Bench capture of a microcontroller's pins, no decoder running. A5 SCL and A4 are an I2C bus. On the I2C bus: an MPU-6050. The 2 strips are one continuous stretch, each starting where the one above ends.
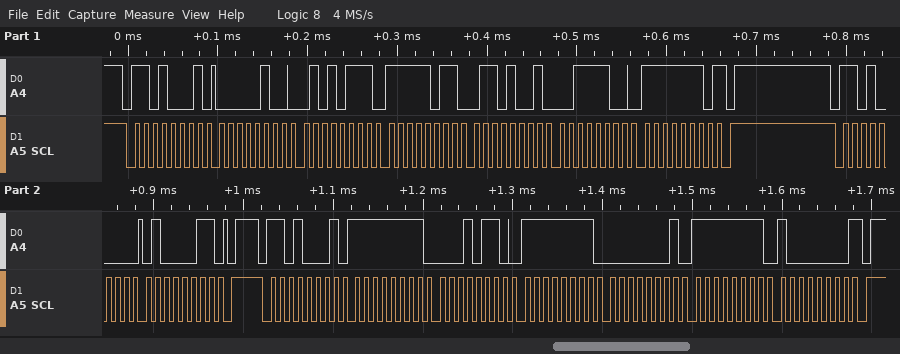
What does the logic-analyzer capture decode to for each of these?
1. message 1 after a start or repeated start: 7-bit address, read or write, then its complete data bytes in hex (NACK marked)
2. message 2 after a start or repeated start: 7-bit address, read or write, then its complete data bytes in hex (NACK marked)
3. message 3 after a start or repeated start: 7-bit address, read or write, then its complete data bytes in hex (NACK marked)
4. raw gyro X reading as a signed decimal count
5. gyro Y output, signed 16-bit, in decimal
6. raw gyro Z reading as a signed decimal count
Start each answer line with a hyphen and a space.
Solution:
- 0x68 read: 04 57 FB 69 3C FE NACK
- 0x68 write: 43
- 0x68 read: FF 16 FF 01 FF 80 NACK
- -234
- -255
- -128
